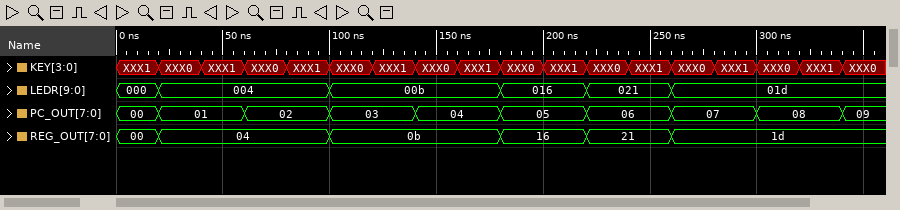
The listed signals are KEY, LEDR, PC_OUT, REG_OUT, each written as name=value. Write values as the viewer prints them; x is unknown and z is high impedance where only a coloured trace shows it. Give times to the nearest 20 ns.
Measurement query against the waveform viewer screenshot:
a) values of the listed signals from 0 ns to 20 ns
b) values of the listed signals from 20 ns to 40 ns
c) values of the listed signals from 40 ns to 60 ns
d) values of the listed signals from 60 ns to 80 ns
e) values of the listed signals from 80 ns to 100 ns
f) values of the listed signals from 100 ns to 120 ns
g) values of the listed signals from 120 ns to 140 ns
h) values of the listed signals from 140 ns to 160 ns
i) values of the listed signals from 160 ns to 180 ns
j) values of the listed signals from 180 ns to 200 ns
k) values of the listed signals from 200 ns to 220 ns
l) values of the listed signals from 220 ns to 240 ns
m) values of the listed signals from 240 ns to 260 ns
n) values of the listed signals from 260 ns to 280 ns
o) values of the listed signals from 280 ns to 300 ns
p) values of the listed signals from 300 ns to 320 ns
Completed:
KEY=XXX1, LEDR=000, PC_OUT=00, REG_OUT=00
KEY=XXX0, LEDR=004, PC_OUT=01, REG_OUT=04
KEY=XXX1, LEDR=004, PC_OUT=01, REG_OUT=04
KEY=XXX0, LEDR=004, PC_OUT=02, REG_OUT=04
KEY=XXX1, LEDR=004, PC_OUT=02, REG_OUT=04
KEY=XXX0, LEDR=00b, PC_OUT=03, REG_OUT=0b
KEY=XXX1, LEDR=00b, PC_OUT=03, REG_OUT=0b
KEY=XXX0, LEDR=00b, PC_OUT=04, REG_OUT=0b
KEY=XXX1, LEDR=00b, PC_OUT=04, REG_OUT=0b
KEY=XXX0, LEDR=016, PC_OUT=05, REG_OUT=16
KEY=XXX1, LEDR=016, PC_OUT=05, REG_OUT=16
KEY=XXX0, LEDR=021, PC_OUT=06, REG_OUT=21
KEY=XXX1, LEDR=021, PC_OUT=06, REG_OUT=21
KEY=XXX0, LEDR=01d, PC_OUT=07, REG_OUT=1d
KEY=XXX1, LEDR=01d, PC_OUT=07, REG_OUT=1d
KEY=XXX0, LEDR=01d, PC_OUT=08, REG_OUT=1d
